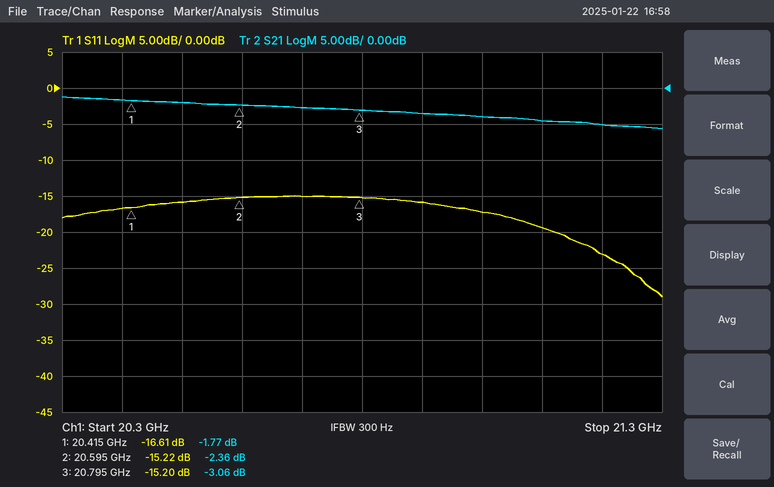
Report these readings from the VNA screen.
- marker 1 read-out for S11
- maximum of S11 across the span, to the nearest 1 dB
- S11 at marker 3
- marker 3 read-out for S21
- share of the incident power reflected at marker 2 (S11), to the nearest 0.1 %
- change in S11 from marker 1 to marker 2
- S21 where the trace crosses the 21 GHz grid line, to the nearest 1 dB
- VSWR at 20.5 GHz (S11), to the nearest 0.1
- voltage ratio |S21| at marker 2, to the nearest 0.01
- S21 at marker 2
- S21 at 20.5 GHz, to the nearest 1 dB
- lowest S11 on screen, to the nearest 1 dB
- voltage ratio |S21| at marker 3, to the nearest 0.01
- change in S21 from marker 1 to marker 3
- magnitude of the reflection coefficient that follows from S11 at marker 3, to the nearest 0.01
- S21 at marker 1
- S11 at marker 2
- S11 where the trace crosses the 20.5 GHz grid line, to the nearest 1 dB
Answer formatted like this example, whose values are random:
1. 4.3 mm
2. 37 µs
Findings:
1. -16.61 dB
2. -15 dB
3. -15.20 dB
4. -3.06 dB
5. 3.0 %
6. 1.39 dB
7. -4 dB
8. 1.4
9. 0.76
10. -2.36 dB
11. -2 dB
12. -29 dB
13. 0.70
14. -1.29 dB
15. 0.17
16. -1.77 dB
17. -15.22 dB
18. -16 dB
